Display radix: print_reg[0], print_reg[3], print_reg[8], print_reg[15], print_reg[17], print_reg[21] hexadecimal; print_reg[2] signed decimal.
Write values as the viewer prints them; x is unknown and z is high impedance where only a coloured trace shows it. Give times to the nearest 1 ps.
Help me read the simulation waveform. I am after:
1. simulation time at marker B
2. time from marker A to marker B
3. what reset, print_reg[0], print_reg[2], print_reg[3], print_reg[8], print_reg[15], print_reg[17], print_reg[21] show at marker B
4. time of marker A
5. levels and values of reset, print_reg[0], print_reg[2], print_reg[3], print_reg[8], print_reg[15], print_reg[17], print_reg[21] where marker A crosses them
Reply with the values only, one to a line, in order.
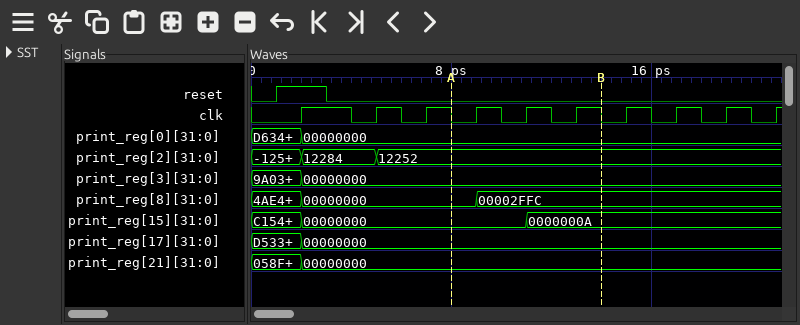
14 ps
6 ps
reset=0, print_reg[0]=00000000, print_reg[2]=12252, print_reg[3]=00000000, print_reg[8]=00002FFC, print_reg[15]=0000000A, print_reg[17]=00000000, print_reg[21]=00000000
8 ps
reset=0, print_reg[0]=00000000, print_reg[2]=12252, print_reg[3]=00000000, print_reg[8]=00000000, print_reg[15]=00000000, print_reg[17]=00000000, print_reg[21]=00000000
